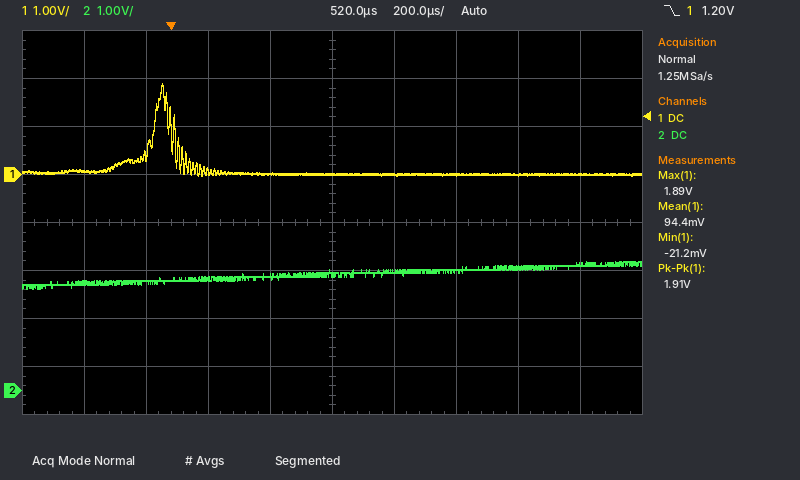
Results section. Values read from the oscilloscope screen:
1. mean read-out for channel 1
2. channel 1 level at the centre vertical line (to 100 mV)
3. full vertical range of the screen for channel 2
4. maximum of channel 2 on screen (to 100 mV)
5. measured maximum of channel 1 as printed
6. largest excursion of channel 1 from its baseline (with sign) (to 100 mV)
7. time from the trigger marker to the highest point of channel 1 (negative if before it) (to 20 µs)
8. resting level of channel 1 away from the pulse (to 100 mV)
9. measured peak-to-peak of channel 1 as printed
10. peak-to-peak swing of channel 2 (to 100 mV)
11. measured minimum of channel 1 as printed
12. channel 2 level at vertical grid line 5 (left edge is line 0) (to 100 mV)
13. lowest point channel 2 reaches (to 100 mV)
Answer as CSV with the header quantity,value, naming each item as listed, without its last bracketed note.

quantity,value
mean read-out for channel 1,94.4 mV
channel 1 level at the centre vertical line,0.0 V
full vertical range of the screen for channel 2,8 V
maximum of channel 2 on screen,2.7 V
measured maximum of channel 1 as printed,1.89 V
largest excursion of channel 1 from its baseline (with sign),+1.9 V
time from the trigger marker to the highest point of channel 1 (negative if before it),-20 µs
resting level of channel 1 away from the pulse,0.0 V
measured peak-to-peak of channel 1 as printed,1.91 V
peak-to-peak swing of channel 2,600 mV
measured minimum of channel 1 as printed,-21.2 mV
channel 2 level at vertical grid line 5 (left edge is line 0),2.4 V
lowest point channel 2 reaches,2.1 V
